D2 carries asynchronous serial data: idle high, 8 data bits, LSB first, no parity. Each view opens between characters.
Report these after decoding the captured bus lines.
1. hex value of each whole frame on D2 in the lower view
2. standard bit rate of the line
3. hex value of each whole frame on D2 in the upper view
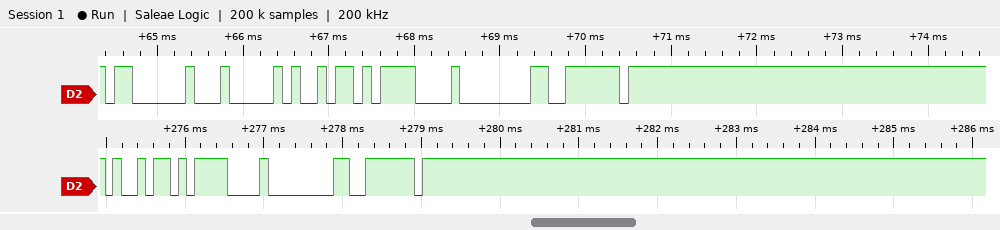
69, 0F, 80, 7E
9600 baud
03, 04, 69, 0F, 80, 7E
